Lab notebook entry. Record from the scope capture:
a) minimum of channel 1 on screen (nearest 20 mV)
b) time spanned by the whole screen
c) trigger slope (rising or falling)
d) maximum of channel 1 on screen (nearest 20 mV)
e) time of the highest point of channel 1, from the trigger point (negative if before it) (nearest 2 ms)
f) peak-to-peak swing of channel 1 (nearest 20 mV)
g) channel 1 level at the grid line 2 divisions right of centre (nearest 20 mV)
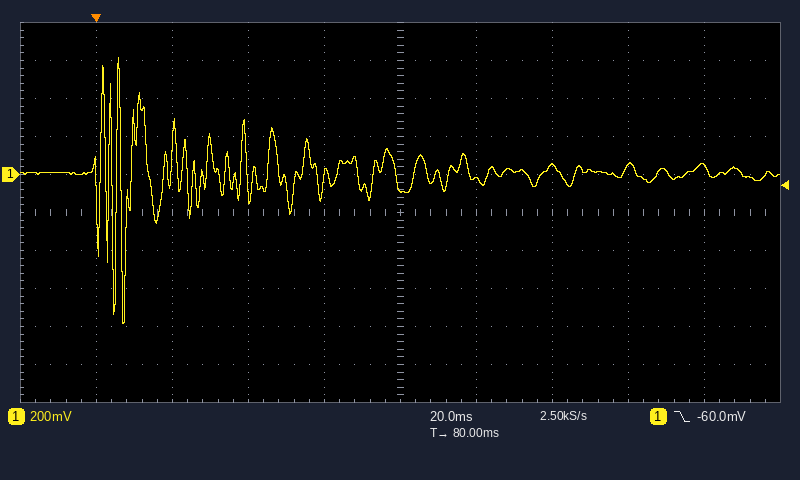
-780 mV
200 ms
falling
620 mV
+6 ms
1.40 V
40 mV
